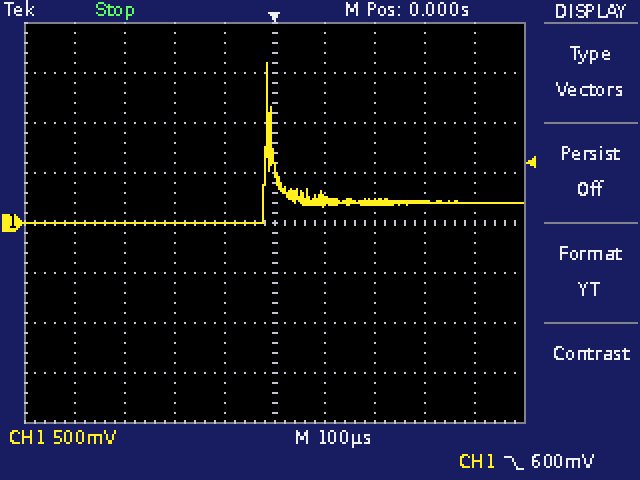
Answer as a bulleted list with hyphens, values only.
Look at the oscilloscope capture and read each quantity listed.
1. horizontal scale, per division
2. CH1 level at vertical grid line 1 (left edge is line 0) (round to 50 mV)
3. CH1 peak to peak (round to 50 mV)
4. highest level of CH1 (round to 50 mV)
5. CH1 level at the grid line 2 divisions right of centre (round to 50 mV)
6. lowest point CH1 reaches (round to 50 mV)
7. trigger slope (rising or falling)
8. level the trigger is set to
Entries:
- 100 µs
- 0 mV
- 1.60 V
- 1.60 V
- 200 mV
- 0 mV
- falling
- 600 mV
